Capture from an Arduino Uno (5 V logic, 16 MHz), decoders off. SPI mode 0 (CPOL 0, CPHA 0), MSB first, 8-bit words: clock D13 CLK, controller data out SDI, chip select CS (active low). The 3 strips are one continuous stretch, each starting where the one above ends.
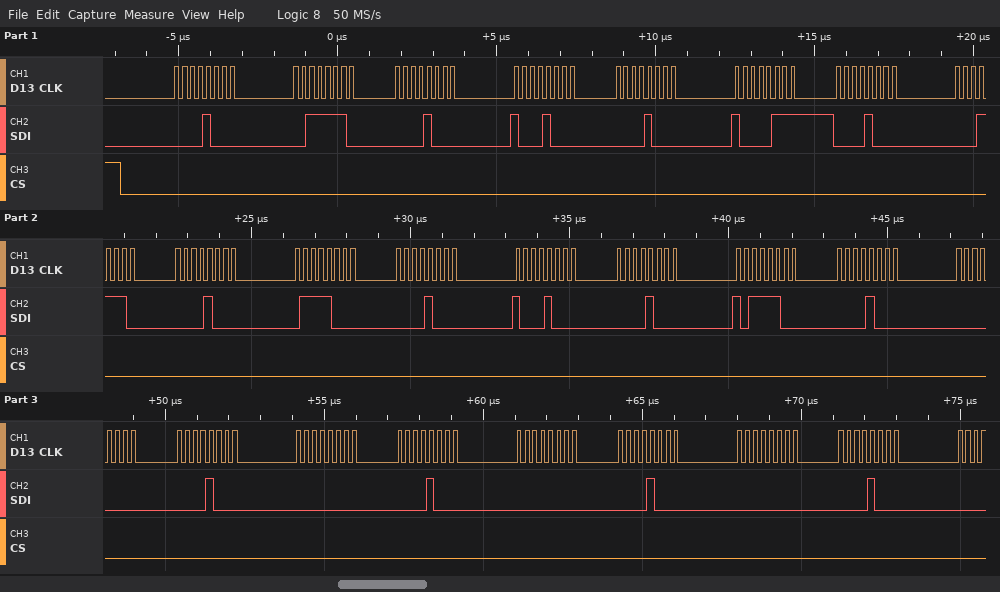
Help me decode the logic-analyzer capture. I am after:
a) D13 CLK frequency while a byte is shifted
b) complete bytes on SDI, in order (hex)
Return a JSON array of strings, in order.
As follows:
["4 MHz", "08 3E 08 88 08 87 08 1E 08 78 08 88 08 BC 08 00 08 00 08 00 08 00 08"]
